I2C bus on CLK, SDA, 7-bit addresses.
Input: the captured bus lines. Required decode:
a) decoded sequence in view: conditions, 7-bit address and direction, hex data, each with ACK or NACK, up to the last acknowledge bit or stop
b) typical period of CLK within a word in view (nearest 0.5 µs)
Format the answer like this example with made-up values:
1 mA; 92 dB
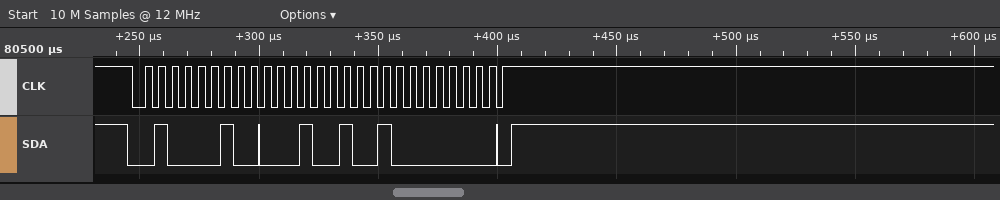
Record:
start, address 21 write ACK, 12 ACK, 80 ACK, stop; 5.5 µs
